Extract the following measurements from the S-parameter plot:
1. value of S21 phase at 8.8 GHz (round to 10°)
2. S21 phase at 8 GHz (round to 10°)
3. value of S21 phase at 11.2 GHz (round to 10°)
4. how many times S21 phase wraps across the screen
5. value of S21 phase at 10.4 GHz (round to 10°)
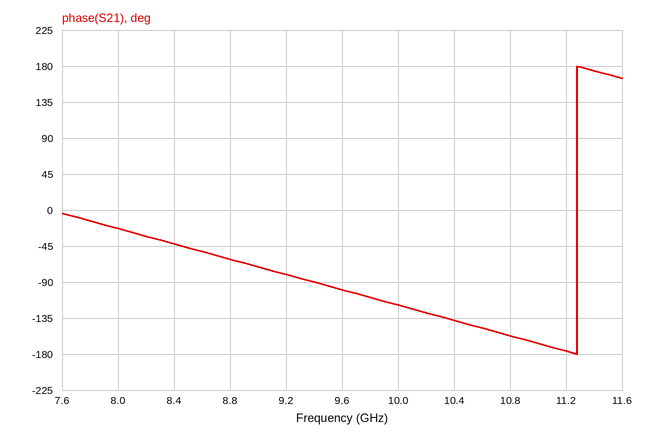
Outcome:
-60°
-20°
-180°
1
-140°
